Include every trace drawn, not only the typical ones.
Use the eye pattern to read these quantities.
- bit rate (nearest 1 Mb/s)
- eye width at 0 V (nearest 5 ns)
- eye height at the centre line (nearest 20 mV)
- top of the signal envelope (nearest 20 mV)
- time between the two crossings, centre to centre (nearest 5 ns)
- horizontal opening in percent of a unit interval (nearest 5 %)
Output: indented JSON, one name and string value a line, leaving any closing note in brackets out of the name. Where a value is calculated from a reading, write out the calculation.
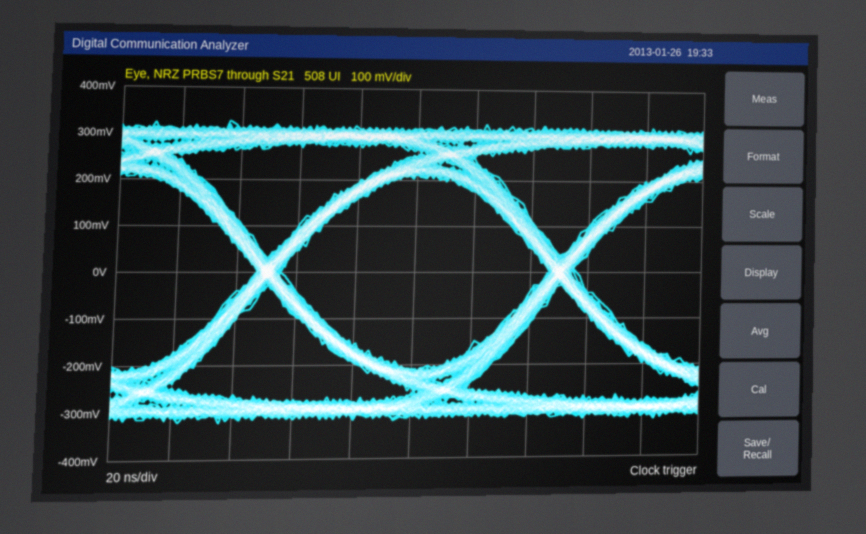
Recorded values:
{
  "bit rate": "10 Mb/s",
  "eye width at 0 V": "90 ns",
  "eye height at the centre line": "420 mV",
  "top of the signal envelope": "320 mV",
  "time between the two crossings, centre to centre": "100 ns",
  "horizontal opening in percent of a unit interval": "90 ns / 100 ns ≈ 90 %"
}
